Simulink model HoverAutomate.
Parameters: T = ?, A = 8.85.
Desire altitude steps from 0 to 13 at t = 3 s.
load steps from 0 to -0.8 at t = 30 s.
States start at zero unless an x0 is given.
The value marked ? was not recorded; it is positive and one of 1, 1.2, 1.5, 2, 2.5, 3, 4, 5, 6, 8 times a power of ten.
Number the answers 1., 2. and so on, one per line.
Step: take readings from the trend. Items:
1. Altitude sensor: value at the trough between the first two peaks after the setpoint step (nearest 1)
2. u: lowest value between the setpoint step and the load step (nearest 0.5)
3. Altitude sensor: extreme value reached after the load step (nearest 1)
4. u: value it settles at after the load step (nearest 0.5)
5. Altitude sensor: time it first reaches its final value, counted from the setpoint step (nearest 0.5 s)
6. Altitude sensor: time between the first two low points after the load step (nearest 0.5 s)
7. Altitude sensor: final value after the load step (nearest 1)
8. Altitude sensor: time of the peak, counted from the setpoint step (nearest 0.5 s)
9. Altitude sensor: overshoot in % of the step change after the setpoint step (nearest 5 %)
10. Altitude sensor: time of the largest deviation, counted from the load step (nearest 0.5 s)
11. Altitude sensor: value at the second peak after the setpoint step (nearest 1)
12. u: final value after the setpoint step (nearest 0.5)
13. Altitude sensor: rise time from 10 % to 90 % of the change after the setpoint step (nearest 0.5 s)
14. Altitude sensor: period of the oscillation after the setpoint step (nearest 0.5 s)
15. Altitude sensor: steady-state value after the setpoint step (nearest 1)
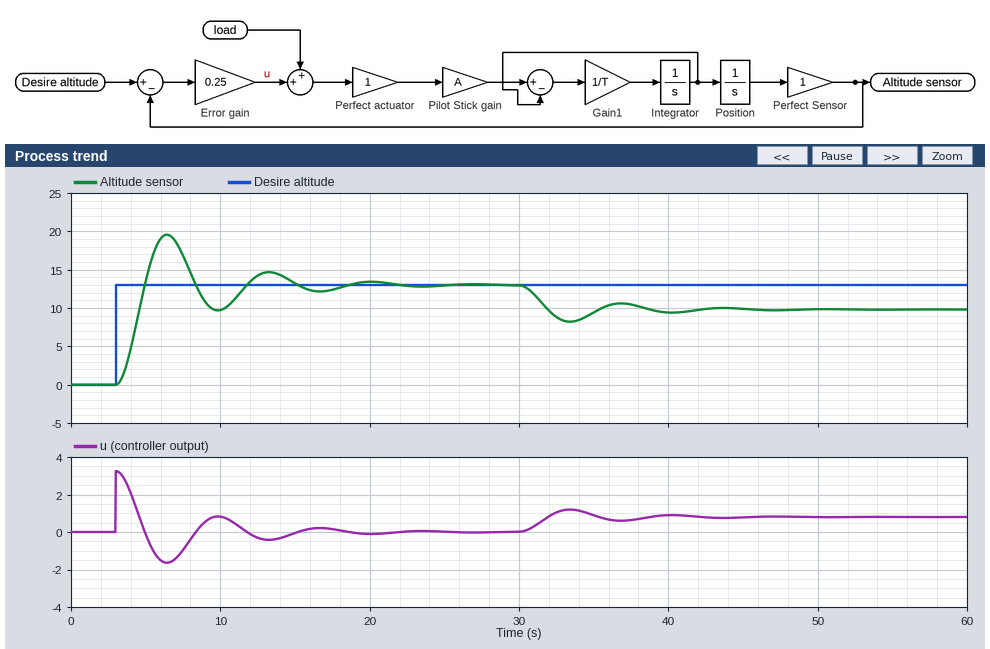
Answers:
1. 10
2. -1.5
3. 8
4. 1.0
5. 2.0 s
6. 7.0 s
7. 10
8. 3.5 s
9. 50 %
10. 3.5 s
11. 15
12. 0.0
13. 1.5 s
14. 7.0 s
15. 13
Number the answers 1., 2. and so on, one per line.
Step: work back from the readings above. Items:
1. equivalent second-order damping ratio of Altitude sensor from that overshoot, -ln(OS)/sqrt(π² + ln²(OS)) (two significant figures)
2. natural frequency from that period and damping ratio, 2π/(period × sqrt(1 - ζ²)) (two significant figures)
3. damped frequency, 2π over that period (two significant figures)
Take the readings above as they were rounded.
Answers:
1. 0.22
2. 0.92 rad/s
3. 0.90 rad/s
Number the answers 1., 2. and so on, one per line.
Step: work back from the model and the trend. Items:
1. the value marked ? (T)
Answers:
1. 2.5
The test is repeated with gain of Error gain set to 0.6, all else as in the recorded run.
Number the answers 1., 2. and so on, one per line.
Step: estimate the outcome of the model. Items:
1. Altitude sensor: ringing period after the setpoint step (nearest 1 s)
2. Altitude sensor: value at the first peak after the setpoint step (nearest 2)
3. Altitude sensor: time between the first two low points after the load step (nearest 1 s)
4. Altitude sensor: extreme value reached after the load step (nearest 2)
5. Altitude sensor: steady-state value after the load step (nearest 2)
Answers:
1. 4 s
2. 22
3. 4 s
4. 10
5. 12
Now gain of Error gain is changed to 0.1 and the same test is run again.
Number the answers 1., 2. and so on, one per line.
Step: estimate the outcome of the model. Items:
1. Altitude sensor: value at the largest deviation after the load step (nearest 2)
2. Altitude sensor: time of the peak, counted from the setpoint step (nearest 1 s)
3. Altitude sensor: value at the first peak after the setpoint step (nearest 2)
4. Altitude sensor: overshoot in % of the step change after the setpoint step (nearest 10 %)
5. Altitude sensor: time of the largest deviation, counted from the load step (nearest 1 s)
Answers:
1. 2
2. 6 s
3. 18
4. 30 %
5. 6 s
